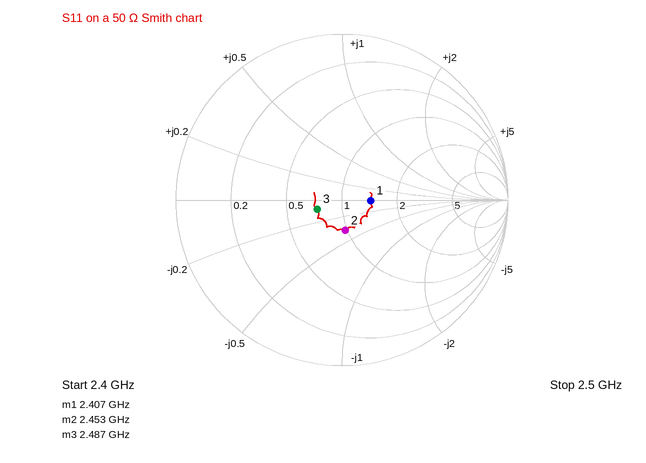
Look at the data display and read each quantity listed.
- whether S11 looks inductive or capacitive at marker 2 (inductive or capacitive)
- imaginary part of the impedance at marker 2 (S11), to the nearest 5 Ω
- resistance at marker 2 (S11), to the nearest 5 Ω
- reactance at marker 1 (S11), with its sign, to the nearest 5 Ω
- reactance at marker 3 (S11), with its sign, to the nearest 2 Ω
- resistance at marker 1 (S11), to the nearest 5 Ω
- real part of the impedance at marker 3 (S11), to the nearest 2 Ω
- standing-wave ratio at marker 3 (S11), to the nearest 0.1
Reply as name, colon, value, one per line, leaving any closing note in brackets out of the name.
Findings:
whether S11 looks inductive or capacitive at marker 2: capacitive
imaginary part of the impedance at marker 2 (S11), to the nearest 5 Ω: -20 Ω
resistance at marker 2 (S11), to the nearest 5 Ω: 50 Ω
reactance at marker 1 (S11), with its sign, to the nearest 5 Ω: 0 Ω
reactance at marker 3 (S11), with its sign, to the nearest 2 Ω: -4 Ω
resistance at marker 1 (S11), to the nearest 5 Ω: 70 Ω
real part of the impedance at marker 3 (S11), to the nearest 2 Ω: 36 Ω
standing-wave ratio at marker 3 (S11), to the nearest 0.1: 1.4
